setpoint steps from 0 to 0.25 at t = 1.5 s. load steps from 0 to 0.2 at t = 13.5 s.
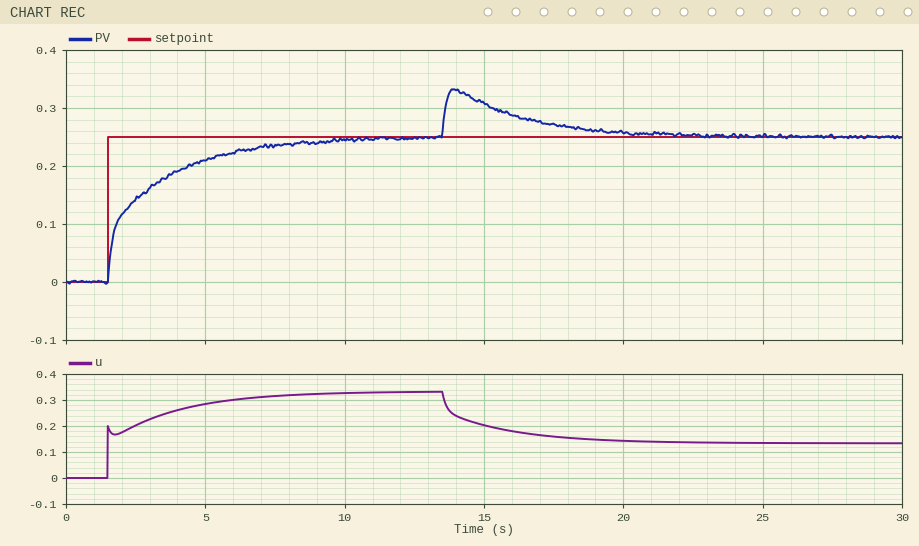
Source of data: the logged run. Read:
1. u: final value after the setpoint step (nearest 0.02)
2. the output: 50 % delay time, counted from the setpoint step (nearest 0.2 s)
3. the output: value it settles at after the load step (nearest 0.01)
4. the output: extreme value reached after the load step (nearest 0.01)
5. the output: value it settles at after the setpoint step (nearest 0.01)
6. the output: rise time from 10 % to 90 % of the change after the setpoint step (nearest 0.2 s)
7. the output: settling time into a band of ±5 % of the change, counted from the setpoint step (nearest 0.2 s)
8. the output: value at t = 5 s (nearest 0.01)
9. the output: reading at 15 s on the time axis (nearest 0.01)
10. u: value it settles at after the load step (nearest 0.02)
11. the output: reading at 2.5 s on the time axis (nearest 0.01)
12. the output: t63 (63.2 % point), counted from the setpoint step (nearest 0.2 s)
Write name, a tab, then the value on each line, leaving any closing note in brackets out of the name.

u: final value after the setpoint step	0.34
the output: 50 % delay time, counted from the setpoint step	0.6 s
the output: value it settles at after the load step	0.25
the output: extreme value reached after the load step	0.33
the output: value it settles at after the setpoint step	0.25
the output: rise time from 10 % to 90 % of the change after the setpoint step	4.6 s
the output: settling time into a band of ±5 % of the change, counted from the setpoint step	6.4 s
the output: value at t = 5 s	0.21
the output: reading at 15 s on the time axis	0.31
u: value it settles at after the load step	0.14
the output: reading at 2.5 s on the time axis	0.14
the output: t63 (63.2 % point), counted from the setpoint step	1.4 s
